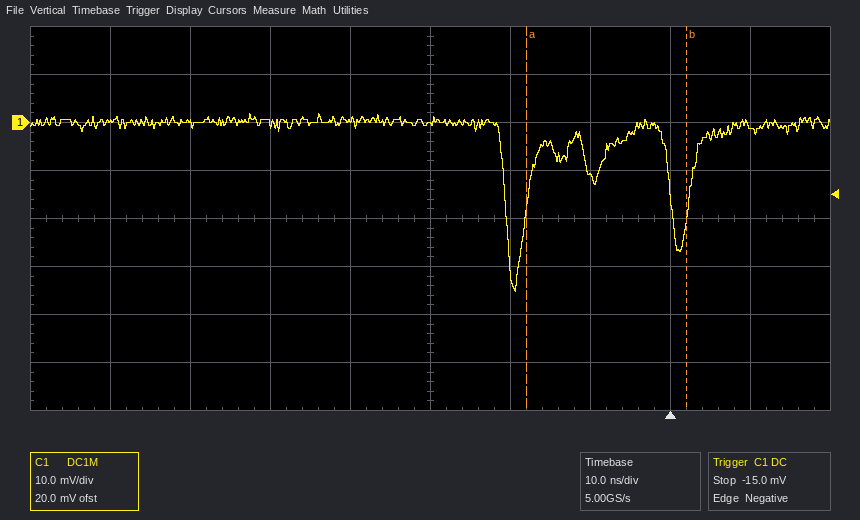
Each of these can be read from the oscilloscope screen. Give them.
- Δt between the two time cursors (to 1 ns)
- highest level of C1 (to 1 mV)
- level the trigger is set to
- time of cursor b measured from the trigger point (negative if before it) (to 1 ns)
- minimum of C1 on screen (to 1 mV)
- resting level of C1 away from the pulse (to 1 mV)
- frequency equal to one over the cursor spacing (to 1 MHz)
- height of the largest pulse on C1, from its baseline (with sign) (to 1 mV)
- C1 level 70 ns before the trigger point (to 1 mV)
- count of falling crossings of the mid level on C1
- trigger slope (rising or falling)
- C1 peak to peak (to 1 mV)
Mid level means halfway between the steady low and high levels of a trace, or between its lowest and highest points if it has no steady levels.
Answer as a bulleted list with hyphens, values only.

- 20 ns
- 2 mV
- -15.0 mV
- +2 ns
- -35 mV
- 0 mV
- 50 MHz
- -35 mV
- 0 mV
- 2
- falling
- 37 mV
